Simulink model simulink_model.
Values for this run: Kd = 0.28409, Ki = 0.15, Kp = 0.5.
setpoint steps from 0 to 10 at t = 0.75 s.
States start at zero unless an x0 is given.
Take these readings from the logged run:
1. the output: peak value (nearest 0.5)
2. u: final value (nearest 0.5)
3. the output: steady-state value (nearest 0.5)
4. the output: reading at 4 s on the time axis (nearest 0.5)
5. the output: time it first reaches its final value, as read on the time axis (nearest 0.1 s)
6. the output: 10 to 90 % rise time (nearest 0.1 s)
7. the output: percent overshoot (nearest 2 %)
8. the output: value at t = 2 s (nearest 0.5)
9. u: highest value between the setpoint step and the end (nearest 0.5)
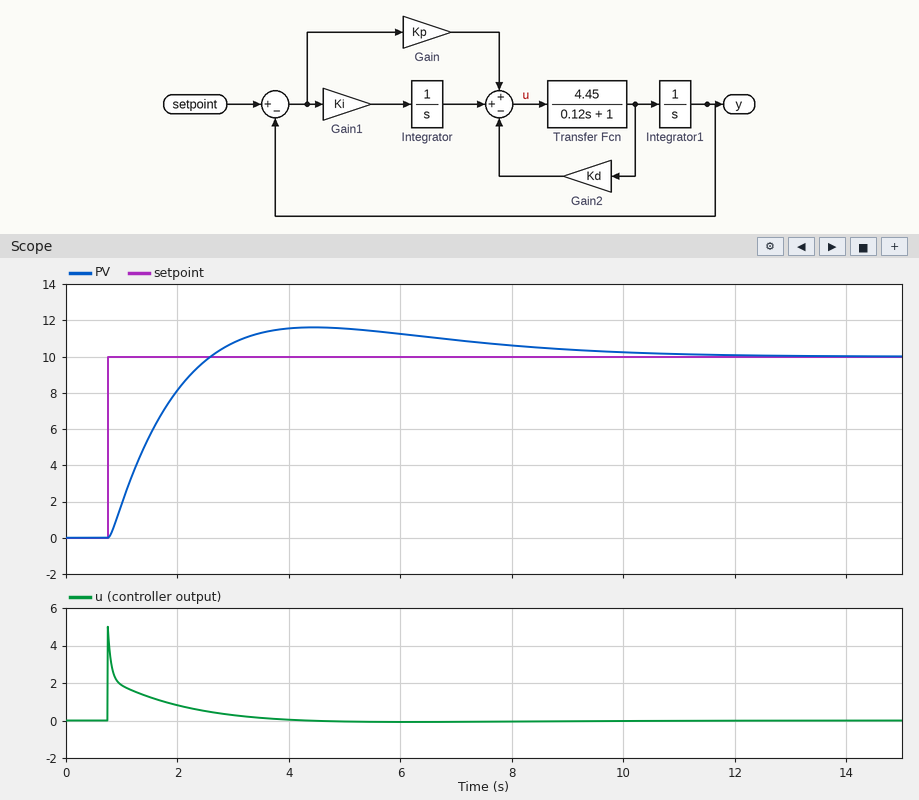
11.5
0.0
10.0
11.5
2.6 s
1.3 s
16 %
8.0
5.0
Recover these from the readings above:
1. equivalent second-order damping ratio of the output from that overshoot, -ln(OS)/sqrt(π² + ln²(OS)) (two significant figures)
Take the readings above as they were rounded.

0.50
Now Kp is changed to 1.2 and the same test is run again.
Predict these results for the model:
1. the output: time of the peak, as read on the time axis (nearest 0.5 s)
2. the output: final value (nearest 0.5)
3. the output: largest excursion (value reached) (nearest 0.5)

3.0 s
10.0
10.5
